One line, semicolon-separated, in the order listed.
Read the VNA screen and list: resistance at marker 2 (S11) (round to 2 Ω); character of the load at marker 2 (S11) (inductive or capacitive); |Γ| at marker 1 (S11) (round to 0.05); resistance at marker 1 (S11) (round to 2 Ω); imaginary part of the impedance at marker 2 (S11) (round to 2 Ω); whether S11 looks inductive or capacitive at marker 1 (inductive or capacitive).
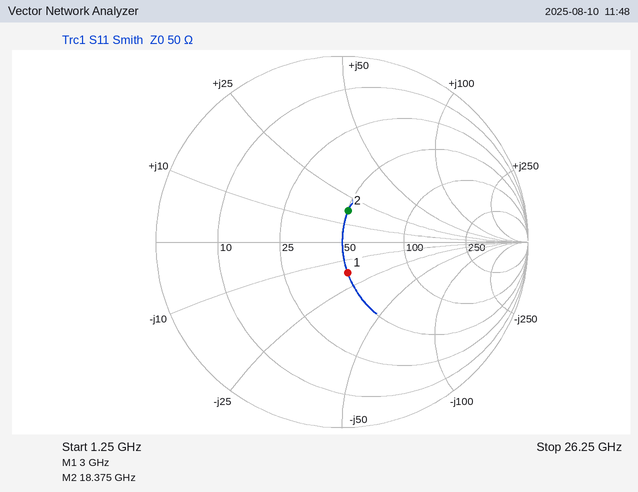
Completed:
50 Ω; inductive; 0.15; 50 Ω; +18 Ω; capacitive
